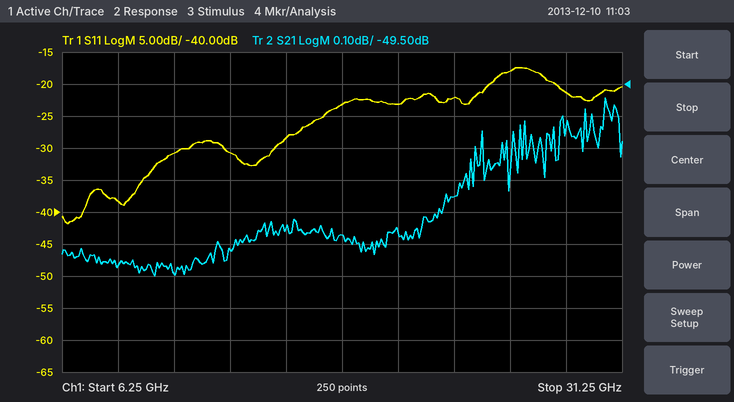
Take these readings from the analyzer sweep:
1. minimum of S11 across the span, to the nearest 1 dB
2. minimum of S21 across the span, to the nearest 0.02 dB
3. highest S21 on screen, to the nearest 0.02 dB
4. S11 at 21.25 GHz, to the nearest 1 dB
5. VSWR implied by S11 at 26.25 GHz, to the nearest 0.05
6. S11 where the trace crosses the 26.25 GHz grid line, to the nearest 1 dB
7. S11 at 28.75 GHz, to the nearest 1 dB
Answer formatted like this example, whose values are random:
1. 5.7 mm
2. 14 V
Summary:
1. -42 dB
2. -50.10 dB
3. -49.54 dB
4. -23 dB
5. 1.30
6. -18 dB
7. -21 dB
